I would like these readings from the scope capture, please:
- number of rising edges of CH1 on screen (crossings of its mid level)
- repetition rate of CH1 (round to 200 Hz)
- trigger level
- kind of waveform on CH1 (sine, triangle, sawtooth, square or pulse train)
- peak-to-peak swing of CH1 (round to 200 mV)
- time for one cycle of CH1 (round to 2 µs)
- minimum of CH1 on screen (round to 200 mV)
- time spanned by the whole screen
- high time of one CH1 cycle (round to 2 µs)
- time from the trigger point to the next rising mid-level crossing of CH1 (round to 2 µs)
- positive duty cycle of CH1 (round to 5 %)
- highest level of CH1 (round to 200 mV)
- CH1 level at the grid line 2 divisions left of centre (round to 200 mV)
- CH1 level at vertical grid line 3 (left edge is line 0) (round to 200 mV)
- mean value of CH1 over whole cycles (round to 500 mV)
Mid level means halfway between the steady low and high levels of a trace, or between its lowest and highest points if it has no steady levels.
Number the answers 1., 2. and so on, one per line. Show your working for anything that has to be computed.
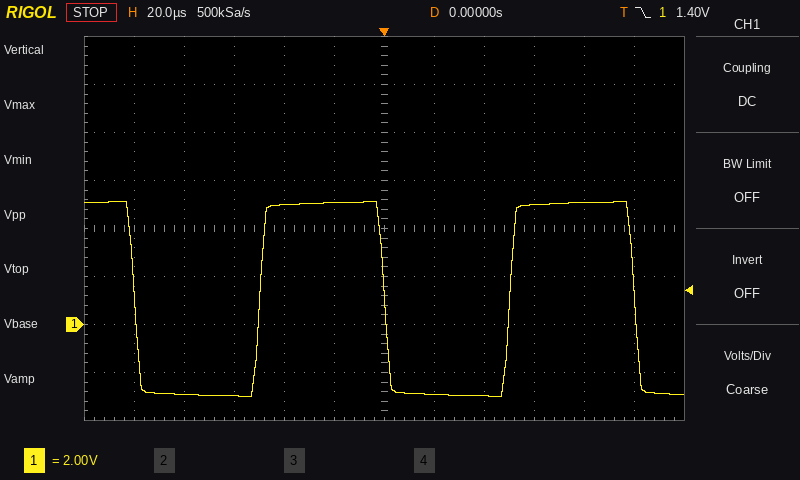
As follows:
1. 2
2. 1 / 100 µs ≈ 10.0 kHz
3. 1.40 V
4. square
5. 5.2 V − (-3.0 V) = 8.2 V
6. 100 µs
7. -3.0 V
8. 240 µs
9. 50 µs
10. 50 µs
11. 50 µs / 100 µs ≈ 50 %
12. 5.2 V
13. 5.0 V
14. -3.0 V
15. -3.0 V + 0.5 × (5.2 V − (-3.0 V)) ≈ 1.10 V, so 1.0 V to the nearest 500 mV
